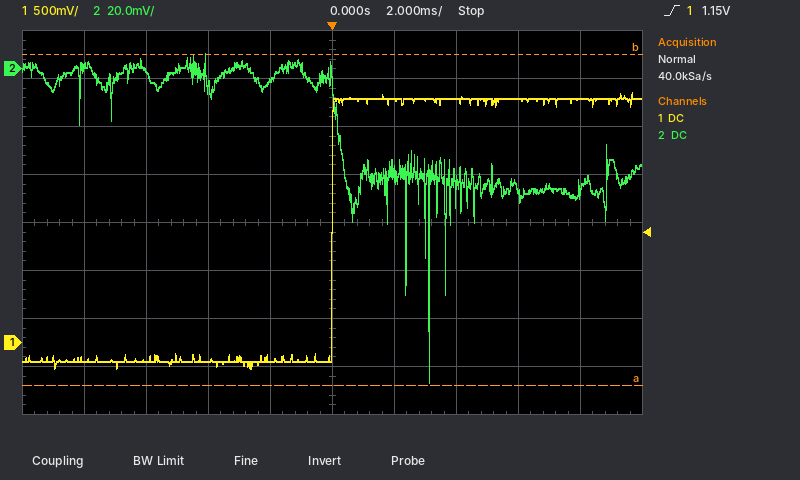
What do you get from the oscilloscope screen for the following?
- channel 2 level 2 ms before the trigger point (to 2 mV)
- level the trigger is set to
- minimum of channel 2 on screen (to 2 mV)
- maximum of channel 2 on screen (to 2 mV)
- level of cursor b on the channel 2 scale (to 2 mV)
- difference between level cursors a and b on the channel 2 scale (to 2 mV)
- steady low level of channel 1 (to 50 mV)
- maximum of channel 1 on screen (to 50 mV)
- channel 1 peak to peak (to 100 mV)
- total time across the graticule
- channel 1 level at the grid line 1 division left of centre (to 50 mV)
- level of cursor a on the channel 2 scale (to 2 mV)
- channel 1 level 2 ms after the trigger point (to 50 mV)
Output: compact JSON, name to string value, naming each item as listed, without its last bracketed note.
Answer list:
{"channel 2 level 2 ms before the trigger point": "-6 mV", "level the trigger is set to": "1.15 V", "minimum of channel 2 on screen": "-130 mV", "maximum of channel 2 on screen": "6 mV", "level of cursor b on the channel 2 scale": "6 mV", "difference between level cursors a and b on the channel 2 scale": "138 mV", "steady low level of channel 1": "-200 mV", "maximum of channel 1 on screen": "2.60 V", "channel 1 peak to peak": "2.90 V", "total time across the graticule": "20 ms", "channel 1 level at the grid line 1 division left of centre": "-150 mV", "level of cursor a on the channel 2 scale": "-132 mV", "channel 1 level 2 ms after the trigger point": "2.55 V"}
